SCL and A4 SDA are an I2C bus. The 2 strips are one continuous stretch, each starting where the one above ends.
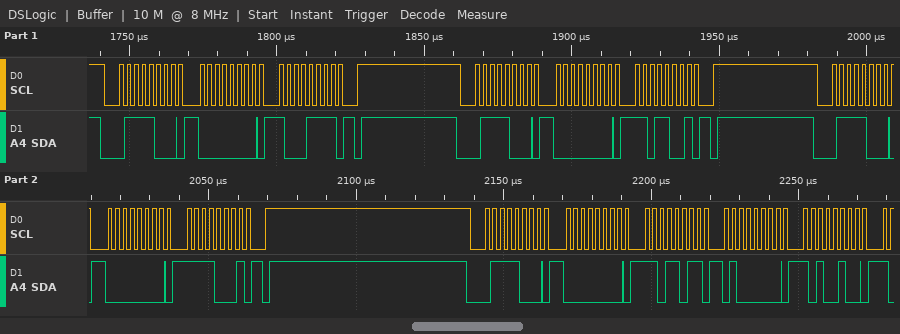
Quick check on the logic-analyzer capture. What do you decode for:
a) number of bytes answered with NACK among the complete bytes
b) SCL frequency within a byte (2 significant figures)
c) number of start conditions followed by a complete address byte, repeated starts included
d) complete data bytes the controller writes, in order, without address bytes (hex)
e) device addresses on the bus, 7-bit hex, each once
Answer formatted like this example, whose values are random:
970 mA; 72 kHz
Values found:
0; 400 kHz; 4; 00 8F 00 D9 00 F1 00 DB 40 A4; 0x3C
